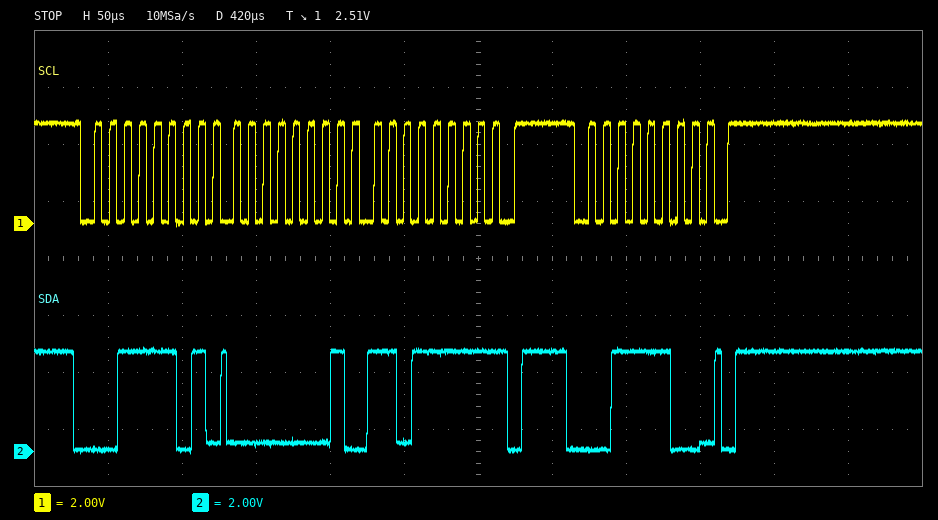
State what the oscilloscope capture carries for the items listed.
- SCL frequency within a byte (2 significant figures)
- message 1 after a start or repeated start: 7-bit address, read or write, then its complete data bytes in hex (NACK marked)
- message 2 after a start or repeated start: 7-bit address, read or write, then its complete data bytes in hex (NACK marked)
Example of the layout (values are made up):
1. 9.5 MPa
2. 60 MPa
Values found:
1. 100 kHz
2. 0x1E read: 01 DF NACK
3. 0x1E write
